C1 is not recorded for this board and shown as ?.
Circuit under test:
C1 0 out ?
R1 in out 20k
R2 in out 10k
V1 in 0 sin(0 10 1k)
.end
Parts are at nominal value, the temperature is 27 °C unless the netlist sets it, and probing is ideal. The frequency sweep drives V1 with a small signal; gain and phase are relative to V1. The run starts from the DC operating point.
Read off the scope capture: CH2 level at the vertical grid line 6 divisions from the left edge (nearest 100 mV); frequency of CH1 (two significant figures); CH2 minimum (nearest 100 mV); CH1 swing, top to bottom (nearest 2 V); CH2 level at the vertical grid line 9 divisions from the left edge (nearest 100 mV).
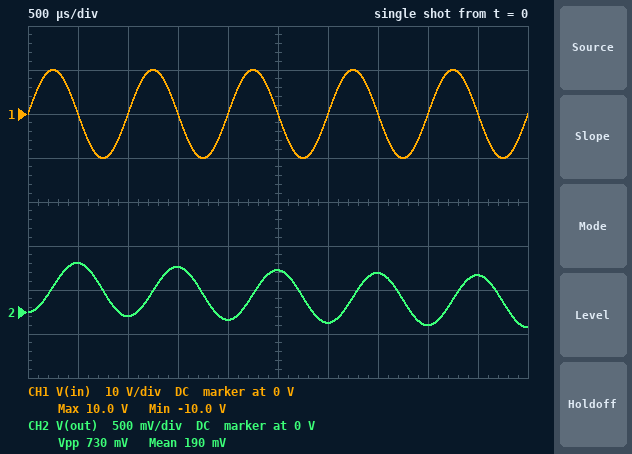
-100 mV
1.0 kHz
-200 mV
20 V
400 mV
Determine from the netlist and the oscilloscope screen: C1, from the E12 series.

820 nF
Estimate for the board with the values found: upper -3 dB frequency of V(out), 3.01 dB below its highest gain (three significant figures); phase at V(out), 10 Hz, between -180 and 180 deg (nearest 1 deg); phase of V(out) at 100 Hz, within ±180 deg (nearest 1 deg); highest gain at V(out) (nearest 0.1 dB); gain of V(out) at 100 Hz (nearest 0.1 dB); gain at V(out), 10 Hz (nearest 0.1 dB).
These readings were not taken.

29.1 Hz
-19 deg
-74 deg
0 dB
-11.1 dB
-0.5 dB
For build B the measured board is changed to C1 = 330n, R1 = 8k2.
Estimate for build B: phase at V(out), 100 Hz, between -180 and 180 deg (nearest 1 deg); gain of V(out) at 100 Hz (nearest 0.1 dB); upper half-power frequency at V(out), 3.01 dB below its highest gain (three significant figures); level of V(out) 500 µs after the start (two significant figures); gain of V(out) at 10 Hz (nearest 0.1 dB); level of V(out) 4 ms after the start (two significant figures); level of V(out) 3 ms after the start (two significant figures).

-43 deg
-2.7 dB
107 Hz
1.8 V
0 dB
-990 mV
-920 mV
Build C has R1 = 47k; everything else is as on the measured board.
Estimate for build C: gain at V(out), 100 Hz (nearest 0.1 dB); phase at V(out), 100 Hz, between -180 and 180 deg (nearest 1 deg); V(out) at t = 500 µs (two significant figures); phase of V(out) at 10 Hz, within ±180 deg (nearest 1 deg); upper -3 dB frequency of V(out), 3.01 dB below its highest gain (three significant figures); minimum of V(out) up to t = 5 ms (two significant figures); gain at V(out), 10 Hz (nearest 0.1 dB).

-12.8 dB
-77 deg
450 mV
-23 deg
23.5 Hz
-120 mV
-0.7 dB
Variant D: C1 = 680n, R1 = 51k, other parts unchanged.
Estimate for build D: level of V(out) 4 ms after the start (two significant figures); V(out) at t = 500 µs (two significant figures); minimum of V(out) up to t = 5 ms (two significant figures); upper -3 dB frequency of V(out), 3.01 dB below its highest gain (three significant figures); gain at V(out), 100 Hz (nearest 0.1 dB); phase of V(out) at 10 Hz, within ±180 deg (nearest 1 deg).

-140 mV
540 mV
-160 mV
28.0 Hz
-11.4 dB
-20 deg
